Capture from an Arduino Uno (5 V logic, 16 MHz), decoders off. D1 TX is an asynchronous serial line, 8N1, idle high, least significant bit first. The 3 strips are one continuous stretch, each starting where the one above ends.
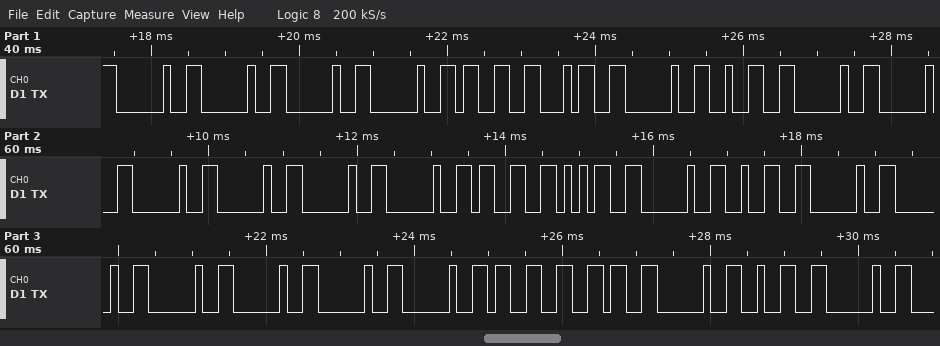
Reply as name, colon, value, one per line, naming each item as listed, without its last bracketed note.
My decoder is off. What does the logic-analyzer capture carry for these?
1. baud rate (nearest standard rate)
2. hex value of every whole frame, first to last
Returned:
baud rate: 9600 baud
hex value of every whole frame, first to last: 20 20 20 20 33 34 20 32 20 20 20 20 20 20 33 35 20 32 20 20 20 20 20 20 33 36 20 32 20
